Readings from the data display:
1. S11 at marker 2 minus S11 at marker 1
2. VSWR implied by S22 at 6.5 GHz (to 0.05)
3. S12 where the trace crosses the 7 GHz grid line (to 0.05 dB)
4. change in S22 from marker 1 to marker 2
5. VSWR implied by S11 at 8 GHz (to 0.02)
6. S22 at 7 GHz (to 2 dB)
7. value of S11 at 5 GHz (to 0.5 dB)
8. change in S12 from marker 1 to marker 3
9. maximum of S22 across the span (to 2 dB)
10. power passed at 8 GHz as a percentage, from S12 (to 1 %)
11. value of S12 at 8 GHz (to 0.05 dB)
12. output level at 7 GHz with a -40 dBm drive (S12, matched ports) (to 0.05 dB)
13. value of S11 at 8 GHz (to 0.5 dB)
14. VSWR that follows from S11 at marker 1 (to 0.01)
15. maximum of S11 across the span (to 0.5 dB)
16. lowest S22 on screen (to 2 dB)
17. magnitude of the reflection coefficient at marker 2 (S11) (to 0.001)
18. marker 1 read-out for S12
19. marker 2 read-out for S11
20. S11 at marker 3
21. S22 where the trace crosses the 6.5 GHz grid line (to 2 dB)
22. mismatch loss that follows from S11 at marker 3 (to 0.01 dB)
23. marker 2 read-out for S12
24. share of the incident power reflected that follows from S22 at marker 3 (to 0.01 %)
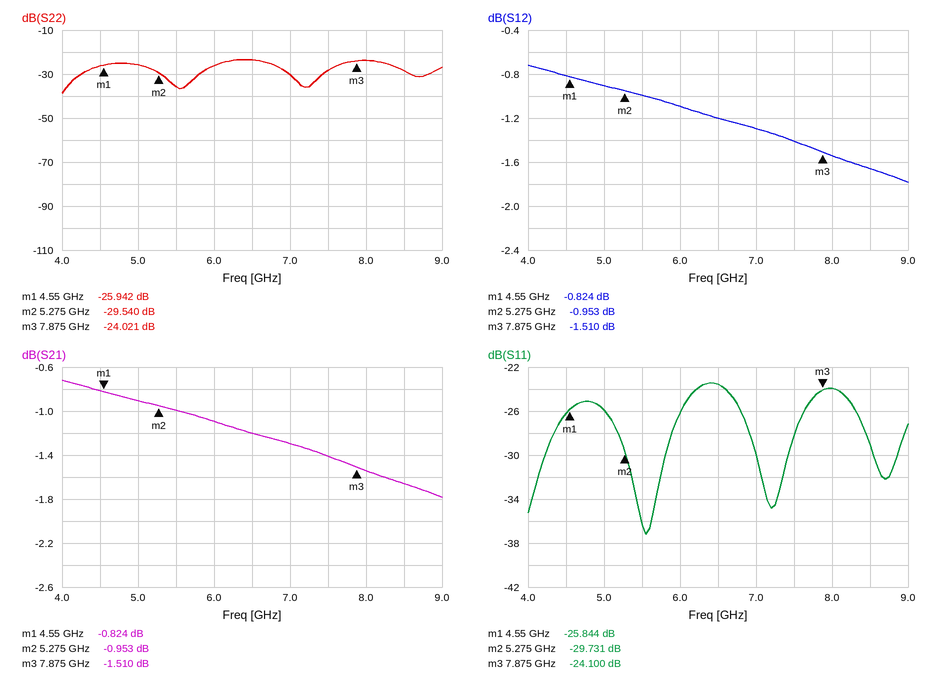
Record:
-3.887 dB
1.15
-1.30 dB
-3.598 dB
1.14
-30 dB
-26.0 dB
-0.686 dB
-24 dB
70 %
-1.55 dB
-41.30 dBm
-24.0 dB
1.11
-23.5 dB
-38 dB
0.033
-0.824 dB
-29.731 dB
-24.100 dB
-24 dB
0.02 dB
-0.953 dB
0.40 %
